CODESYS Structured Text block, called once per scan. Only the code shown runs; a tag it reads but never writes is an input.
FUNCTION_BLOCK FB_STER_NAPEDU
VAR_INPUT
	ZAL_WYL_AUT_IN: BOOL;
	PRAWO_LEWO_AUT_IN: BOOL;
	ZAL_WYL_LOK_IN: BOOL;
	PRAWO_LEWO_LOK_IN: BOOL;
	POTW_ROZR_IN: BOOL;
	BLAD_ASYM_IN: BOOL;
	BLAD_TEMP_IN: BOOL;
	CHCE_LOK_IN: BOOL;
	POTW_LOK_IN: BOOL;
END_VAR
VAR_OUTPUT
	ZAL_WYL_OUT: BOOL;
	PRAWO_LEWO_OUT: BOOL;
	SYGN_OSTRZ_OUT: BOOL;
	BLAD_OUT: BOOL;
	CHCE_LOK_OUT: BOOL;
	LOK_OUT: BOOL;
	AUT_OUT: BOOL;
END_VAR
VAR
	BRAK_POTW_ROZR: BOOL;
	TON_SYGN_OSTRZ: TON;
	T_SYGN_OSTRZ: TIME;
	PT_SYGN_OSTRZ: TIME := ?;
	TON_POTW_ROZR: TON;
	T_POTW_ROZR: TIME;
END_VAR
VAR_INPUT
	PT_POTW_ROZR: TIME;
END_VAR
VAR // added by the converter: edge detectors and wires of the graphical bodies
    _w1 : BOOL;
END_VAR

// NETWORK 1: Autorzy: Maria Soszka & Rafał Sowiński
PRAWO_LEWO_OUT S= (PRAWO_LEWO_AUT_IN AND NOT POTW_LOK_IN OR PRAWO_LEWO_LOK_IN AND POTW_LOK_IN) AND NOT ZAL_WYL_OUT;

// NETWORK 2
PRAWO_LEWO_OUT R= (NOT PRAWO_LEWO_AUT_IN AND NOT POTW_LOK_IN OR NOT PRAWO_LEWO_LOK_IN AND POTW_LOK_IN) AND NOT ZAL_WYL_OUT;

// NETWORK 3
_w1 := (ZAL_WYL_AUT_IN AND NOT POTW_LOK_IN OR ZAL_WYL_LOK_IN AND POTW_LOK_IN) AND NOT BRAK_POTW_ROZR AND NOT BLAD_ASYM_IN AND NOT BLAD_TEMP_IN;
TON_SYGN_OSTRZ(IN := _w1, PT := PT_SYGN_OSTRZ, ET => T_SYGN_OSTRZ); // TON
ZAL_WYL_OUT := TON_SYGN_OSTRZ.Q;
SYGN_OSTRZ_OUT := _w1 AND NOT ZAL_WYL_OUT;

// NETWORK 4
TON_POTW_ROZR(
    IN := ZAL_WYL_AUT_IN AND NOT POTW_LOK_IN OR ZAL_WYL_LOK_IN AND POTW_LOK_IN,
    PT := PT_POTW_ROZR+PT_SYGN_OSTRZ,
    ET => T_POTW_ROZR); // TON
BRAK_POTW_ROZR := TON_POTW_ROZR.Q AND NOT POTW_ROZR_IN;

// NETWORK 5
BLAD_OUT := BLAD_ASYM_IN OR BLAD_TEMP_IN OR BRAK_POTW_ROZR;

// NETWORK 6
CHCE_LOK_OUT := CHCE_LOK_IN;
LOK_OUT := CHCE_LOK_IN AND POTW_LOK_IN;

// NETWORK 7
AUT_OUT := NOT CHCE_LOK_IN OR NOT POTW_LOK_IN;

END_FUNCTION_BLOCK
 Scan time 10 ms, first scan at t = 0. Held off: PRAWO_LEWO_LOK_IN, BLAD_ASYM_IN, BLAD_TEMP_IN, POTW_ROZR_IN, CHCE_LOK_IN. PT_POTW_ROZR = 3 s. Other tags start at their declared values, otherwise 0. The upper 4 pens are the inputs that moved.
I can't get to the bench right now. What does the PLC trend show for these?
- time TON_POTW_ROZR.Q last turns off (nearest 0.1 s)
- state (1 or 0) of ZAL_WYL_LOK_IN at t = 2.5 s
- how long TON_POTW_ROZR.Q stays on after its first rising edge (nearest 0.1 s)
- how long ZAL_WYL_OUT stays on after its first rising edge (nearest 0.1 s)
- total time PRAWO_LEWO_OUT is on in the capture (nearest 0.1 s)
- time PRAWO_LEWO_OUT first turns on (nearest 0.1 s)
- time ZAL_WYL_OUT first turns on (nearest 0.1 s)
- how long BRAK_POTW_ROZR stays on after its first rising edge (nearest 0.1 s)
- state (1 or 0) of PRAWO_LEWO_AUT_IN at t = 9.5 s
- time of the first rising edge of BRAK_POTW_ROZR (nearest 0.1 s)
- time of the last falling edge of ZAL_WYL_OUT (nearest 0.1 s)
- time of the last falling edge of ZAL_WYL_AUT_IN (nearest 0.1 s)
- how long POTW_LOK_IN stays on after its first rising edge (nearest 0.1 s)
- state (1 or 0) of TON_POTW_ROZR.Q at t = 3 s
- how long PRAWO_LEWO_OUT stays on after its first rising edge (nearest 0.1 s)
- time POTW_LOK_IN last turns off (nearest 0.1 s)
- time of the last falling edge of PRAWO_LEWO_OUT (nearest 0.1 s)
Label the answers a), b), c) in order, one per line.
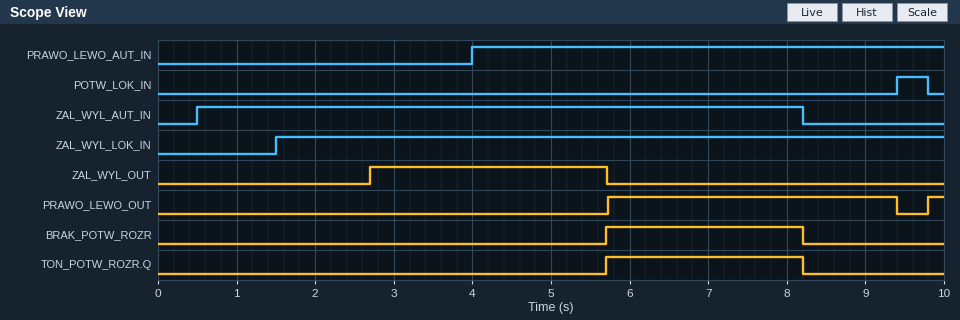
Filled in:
a) 8.2 s
b) 1
c) 2.5 s
d) 3.0 s
e) 3.9 s
f) 5.7 s
g) 2.7 s
h) 2.5 s
i) 1
j) 5.7 s
k) 5.7 s
l) 8.2 s
m) 0.4 s
n) 0
o) 3.7 s
p) 9.8 s
q) 9.4 s
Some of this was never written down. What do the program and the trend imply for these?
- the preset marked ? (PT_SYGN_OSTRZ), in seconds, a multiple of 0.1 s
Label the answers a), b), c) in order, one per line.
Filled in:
a) 2.2 s
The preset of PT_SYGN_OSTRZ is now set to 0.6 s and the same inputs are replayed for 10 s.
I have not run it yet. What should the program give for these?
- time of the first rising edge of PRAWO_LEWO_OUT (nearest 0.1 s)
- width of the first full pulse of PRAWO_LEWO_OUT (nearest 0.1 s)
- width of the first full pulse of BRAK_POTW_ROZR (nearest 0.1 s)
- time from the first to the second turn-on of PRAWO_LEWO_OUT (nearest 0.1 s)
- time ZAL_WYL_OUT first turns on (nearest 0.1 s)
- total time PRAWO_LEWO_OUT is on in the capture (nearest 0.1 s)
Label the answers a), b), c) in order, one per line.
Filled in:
a) 4.1 s
b) 5.3 s
c) 4.1 s
d) 5.7 s
e) 1.1 s
f) 5.5 s
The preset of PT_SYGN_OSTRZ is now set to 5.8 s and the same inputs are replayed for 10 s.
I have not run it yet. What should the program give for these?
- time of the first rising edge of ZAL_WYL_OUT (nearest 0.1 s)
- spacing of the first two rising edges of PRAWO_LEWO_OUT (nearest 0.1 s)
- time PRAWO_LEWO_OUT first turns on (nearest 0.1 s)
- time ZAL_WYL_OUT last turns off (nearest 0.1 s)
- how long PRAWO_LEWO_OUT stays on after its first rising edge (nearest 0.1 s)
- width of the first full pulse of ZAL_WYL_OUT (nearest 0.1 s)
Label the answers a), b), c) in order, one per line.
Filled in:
a) 6.3 s
b) 5.8 s
c) 4.0 s
d) 8.2 s
e) 5.4 s
f) 1.9 s
